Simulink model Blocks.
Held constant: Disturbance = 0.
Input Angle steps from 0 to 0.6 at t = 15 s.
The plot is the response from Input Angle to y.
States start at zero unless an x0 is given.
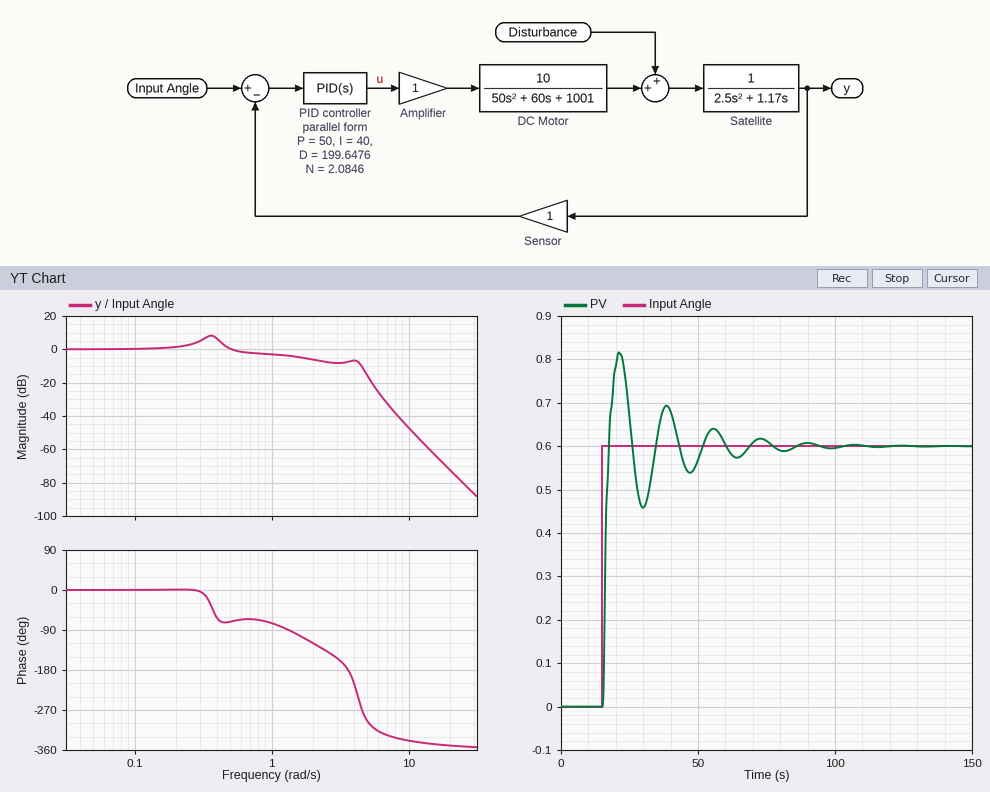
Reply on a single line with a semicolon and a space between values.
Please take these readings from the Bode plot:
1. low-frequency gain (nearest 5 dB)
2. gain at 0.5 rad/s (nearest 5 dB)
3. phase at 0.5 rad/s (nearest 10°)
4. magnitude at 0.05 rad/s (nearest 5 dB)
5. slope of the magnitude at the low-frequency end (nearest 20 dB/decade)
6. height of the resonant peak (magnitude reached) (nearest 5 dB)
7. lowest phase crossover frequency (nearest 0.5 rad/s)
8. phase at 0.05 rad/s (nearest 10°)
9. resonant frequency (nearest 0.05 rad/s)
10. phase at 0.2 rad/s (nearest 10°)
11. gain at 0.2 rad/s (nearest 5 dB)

0 dB; 0 dB; -70°; 0 dB; 0 dB/decade; 10 dB; 3.5 rad/s; 0°; 0.35 rad/s; 0°; 0 dB
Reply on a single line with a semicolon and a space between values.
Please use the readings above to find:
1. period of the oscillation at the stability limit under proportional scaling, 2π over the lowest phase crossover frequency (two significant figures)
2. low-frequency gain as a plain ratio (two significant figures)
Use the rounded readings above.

1.8 s; 1.0
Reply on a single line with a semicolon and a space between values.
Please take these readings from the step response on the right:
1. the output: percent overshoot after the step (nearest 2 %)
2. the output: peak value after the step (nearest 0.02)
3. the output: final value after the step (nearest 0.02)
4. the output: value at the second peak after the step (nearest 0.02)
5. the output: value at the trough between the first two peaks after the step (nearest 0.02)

36 %; 0.82; 0.60; 0.70; 0.46
